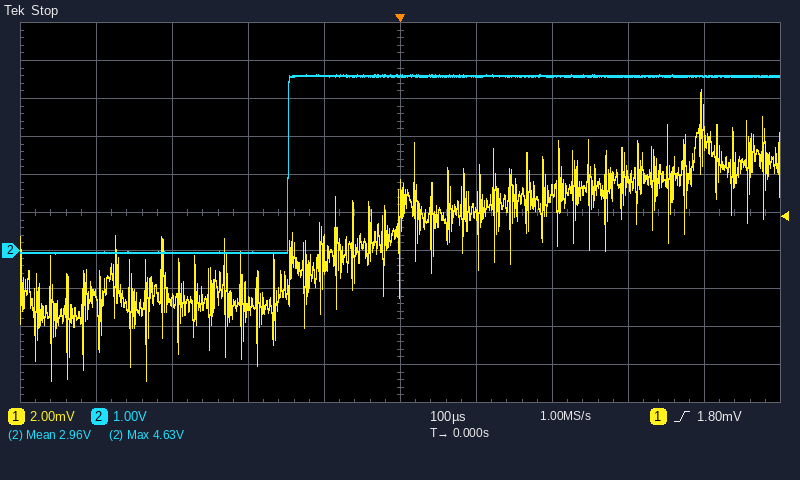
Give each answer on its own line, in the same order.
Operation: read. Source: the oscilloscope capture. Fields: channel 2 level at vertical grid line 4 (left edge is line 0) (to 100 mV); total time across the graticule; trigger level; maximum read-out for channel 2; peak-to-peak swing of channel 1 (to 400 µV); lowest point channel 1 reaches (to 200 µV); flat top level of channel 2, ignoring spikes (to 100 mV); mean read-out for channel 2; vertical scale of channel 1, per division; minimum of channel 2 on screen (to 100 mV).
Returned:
4.6 V
1 ms
1.80 mV
4.63 V
15.2 mV
-6.8 mV
4.6 V
2.96 V
2 mV
-100 mV
